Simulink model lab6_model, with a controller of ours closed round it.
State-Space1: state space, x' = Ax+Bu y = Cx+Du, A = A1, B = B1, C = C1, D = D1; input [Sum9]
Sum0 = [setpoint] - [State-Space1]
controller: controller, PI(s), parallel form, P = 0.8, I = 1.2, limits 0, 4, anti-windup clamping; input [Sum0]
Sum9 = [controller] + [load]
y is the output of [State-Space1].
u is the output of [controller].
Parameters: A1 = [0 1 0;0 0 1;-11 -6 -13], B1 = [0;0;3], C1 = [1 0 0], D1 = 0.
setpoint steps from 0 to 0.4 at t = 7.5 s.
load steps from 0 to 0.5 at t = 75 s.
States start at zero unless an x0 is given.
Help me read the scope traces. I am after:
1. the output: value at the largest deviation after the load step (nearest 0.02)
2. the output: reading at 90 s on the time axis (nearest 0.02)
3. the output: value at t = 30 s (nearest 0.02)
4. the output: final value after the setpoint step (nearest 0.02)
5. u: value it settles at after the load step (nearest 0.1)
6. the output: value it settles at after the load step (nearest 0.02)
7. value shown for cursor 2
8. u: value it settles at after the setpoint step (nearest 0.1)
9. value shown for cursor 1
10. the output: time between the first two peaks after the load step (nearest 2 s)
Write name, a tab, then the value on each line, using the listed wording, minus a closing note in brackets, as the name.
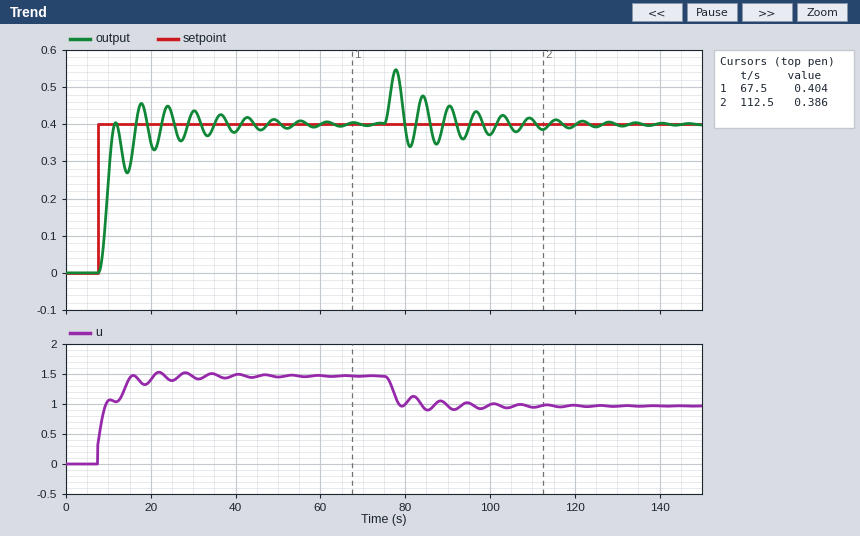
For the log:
the output: value at the largest deviation after the load step	0.54
the output: reading at 90 s on the time axis	0.44
the output: value at t = 30 s	0.44
the output: final value after the setpoint step	0.40
u: value it settles at after the load step	1.0
the output: value it settles at after the load step	0.40
value shown for cursor 2	0.386
u: value it settles at after the setpoint step	1.5
value shown for cursor 1	0.404
the output: time between the first two peaks after the load step	6 s
